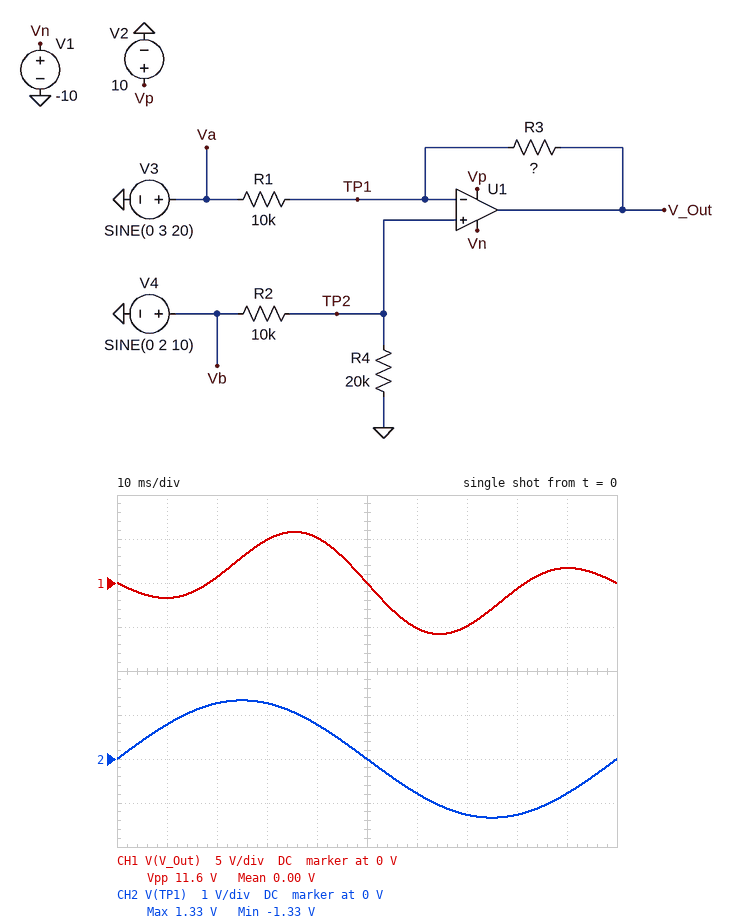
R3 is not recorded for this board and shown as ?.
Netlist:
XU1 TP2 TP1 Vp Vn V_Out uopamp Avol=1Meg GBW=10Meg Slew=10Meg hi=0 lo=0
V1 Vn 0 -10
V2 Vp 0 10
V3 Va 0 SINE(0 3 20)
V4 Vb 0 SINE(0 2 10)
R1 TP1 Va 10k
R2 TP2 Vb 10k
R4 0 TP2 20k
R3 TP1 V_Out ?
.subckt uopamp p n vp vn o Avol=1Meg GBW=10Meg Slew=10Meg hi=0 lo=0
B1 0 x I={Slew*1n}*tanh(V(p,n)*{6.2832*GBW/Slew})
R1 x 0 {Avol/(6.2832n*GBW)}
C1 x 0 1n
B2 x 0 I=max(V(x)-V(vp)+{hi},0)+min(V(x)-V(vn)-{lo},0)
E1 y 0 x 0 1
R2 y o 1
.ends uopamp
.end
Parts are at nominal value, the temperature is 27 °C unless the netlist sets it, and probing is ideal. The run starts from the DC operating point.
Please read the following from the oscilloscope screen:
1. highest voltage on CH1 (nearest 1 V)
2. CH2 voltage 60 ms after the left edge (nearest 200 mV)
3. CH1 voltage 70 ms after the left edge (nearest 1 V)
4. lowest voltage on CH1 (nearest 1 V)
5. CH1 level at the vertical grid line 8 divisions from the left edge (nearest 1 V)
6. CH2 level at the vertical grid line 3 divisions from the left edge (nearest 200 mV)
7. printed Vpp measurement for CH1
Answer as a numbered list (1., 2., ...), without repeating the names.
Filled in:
1. 6 V
2. -800 mV
3. -5 V
4. -6 V
5. -1 V
6. 1.2 V
7. 11.6 V
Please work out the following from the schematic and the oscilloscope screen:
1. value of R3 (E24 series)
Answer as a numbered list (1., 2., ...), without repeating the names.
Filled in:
1. 12 kΩ
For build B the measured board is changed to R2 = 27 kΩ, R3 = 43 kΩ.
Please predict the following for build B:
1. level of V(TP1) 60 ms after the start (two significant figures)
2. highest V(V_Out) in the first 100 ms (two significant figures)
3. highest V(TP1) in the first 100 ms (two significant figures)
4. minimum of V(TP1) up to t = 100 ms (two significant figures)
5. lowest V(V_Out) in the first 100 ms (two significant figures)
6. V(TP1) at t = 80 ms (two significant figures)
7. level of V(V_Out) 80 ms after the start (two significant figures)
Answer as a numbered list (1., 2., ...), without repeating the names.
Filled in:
1. 430 mV
2. 10 V
3. 850 mV
4. -850 mV
5. -10 V
6. -810 mV
7. 3.3 V
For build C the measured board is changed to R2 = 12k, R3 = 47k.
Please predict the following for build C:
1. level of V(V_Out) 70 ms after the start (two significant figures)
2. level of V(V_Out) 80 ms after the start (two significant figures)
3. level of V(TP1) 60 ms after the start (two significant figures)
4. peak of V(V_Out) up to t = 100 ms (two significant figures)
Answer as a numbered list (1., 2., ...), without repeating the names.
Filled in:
1. -10 V
2. 1.5 V
3. 600 mV
4. 10 V
